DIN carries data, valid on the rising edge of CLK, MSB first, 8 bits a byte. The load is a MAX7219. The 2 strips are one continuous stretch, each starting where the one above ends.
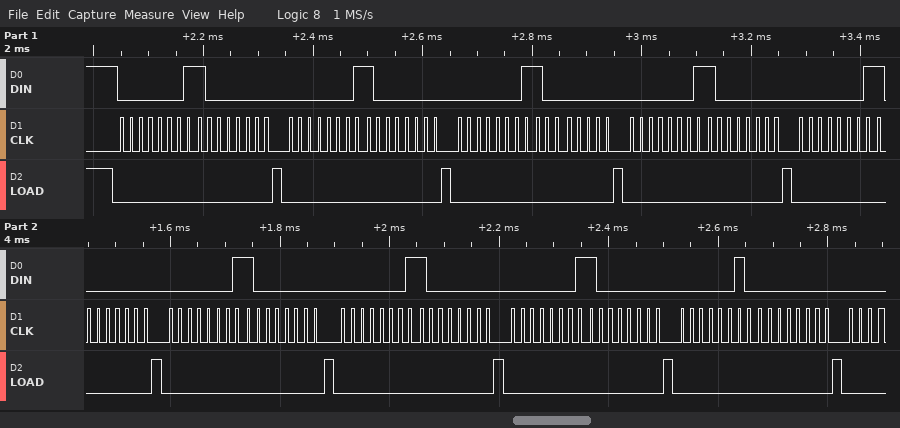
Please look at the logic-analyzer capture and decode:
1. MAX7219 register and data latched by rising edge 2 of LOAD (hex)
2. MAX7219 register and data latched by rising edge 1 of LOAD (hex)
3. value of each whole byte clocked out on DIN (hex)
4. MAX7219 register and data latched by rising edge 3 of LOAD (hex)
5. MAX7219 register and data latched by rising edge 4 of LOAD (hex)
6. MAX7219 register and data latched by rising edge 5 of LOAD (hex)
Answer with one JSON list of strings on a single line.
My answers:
["register 0x1, data 0x80", "register 0x1, data 0x80", "0x01 0x80 0x01 0x80 0x01 0x80 0x01 0x80 0x01 0x80 0x01 0x80 0x01 0x80 0x01 0x80 0x02 0x00", "register 0x1, data 0x80", "register 0x1, data 0x80", "register 0x1, data 0x80"]
